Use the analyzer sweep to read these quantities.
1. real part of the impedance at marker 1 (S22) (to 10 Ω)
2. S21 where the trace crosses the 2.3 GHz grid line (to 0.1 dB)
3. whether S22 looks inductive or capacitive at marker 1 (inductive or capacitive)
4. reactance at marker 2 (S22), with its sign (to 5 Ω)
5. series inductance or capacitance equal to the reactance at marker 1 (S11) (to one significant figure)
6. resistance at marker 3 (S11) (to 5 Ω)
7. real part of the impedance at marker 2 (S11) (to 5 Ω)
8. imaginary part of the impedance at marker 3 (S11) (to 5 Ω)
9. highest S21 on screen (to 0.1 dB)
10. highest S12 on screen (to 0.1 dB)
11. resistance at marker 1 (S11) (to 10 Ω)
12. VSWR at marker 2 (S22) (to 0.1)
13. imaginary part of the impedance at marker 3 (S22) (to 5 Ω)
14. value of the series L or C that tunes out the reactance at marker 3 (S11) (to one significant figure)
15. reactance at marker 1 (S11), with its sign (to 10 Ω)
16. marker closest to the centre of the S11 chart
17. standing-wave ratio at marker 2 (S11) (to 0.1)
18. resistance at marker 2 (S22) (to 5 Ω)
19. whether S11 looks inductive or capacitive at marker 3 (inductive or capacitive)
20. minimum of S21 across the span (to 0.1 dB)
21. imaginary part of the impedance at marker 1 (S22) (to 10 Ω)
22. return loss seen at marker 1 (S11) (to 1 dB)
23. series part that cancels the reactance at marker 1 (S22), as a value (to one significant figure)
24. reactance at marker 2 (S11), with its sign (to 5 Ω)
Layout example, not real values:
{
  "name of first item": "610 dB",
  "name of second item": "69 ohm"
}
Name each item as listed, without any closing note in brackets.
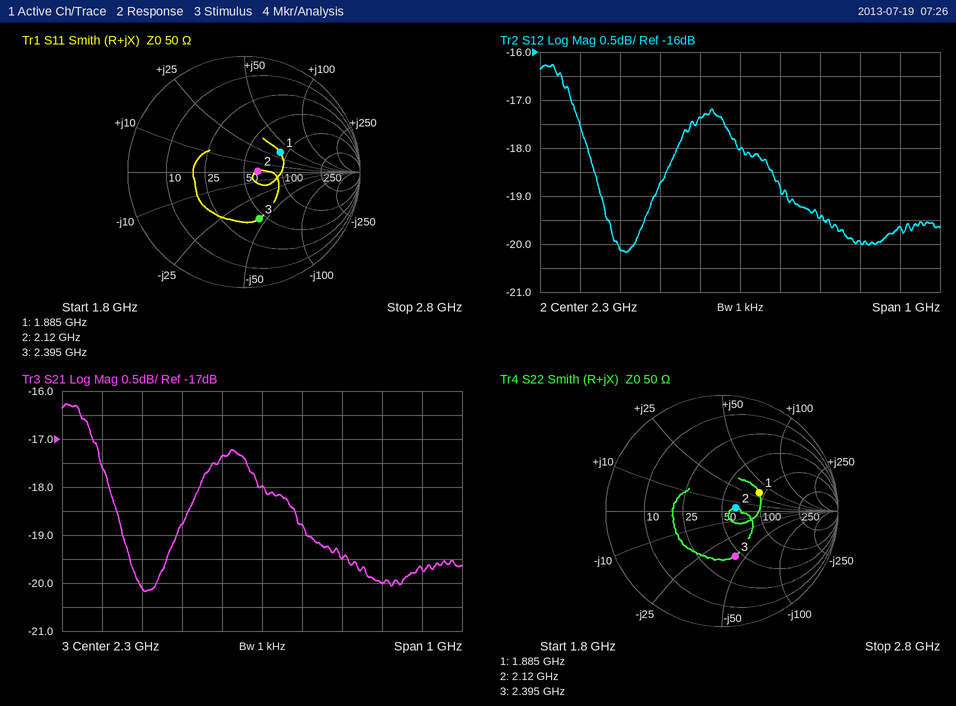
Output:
{
  "real part of the impedance at marker 1 (S22)": "90 Ω",
  "S21 where the trace crosses the 2.3 GHz grid line": "-18.0 dB",
  "whether S22 looks inductive or capacitive at marker 1": "inductive",
  "reactance at marker 2 (S22), with its sign": "+5 Ω",
  "series inductance or capacitance equal to the reactance at marker 1 (S11)": "3 nH",
  "resistance at marker 3 (S11)": "45 Ω",
  "real part of the impedance at marker 2 (S11)": "65 Ω",
  "imaginary part of the impedance at marker 3 (S11)": "-45 Ω",
  "highest S21 on screen": "-16.3 dB",
  "highest S12 on screen": "-16.3 dB",
  "resistance at marker 1 (S11)": "90 Ω",
  "VSWR at marker 2 (S22)": "1.3",
  "imaginary part of the impedance at marker 3 (S22)": "-40 Ω",
  "value of the series L or C that tunes out the reactance at marker 3 (S11)": "3 nH",
  "reactance at marker 1 (S11), with its sign": "+30 Ω",
  "marker closest to the centre of the S11 chart": "marker 2",
  "standing-wave ratio at marker 2 (S11)": "1.3",
  "resistance at marker 2 (S22)": "65 Ω",
  "whether S11 looks inductive or capacitive at marker 3": "capacitive",
  "minimum of S21 across the span": "-20.2 dB",
  "imaginary part of the impedance at marker 1 (S22)": "+30 Ω",
  "return loss seen at marker 1 (S11)": "9 dB",
  "series part that cancels the reactance at marker 1 (S22), as a value": "3 pF",
  "reactance at marker 2 (S11), with its sign": "0 Ω"
}
